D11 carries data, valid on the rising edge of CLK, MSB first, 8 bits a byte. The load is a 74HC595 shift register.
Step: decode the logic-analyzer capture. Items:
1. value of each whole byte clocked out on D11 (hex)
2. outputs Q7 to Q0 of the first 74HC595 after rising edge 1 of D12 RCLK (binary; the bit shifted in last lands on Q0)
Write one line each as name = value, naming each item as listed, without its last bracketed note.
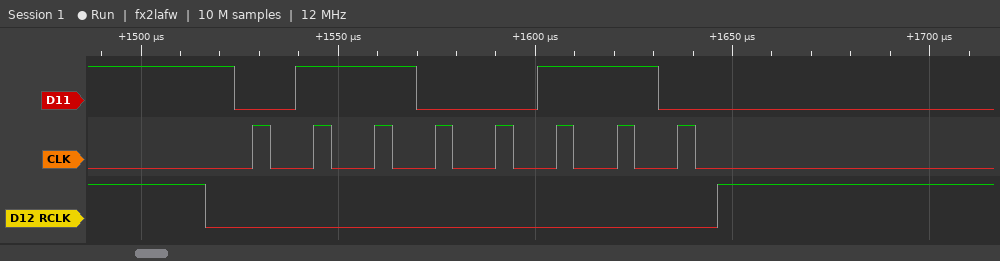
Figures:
value of each whole byte clocked out on D11 = 0x66
outputs Q7 to Q0 of the first 74HC595 after rising edge 1 of D12 RCLK = 01100110
